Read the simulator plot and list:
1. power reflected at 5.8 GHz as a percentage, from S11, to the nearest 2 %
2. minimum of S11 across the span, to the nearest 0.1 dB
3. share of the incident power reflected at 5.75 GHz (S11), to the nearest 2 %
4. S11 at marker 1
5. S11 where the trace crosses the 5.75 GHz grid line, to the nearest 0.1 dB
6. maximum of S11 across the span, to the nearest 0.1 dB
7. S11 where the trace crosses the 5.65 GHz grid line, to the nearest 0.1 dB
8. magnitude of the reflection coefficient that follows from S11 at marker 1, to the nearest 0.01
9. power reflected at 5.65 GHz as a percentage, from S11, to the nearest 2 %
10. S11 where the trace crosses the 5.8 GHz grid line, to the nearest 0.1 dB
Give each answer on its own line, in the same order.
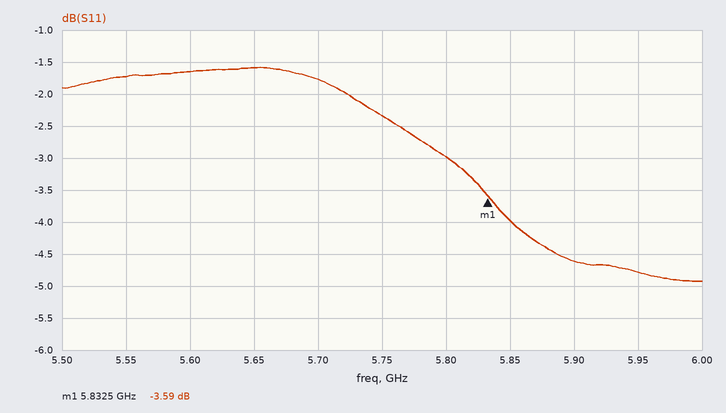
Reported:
50 %
-4.9 dB
58 %
-3.59 dB
-2.3 dB
-1.6 dB
-1.6 dB
0.66
70 %
-3.0 dB
